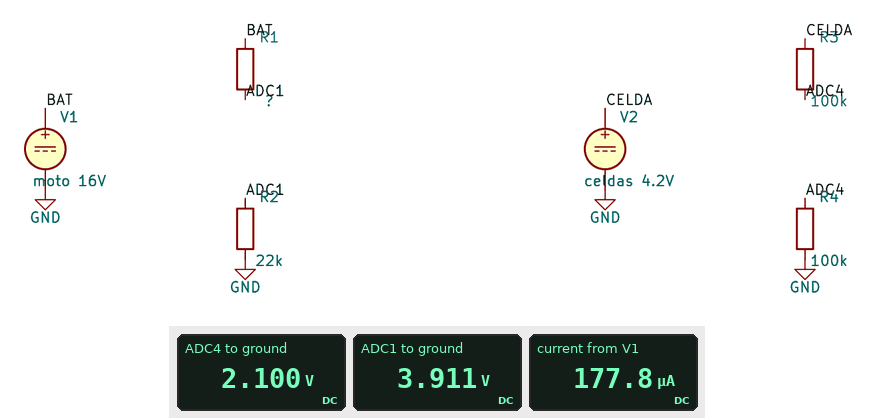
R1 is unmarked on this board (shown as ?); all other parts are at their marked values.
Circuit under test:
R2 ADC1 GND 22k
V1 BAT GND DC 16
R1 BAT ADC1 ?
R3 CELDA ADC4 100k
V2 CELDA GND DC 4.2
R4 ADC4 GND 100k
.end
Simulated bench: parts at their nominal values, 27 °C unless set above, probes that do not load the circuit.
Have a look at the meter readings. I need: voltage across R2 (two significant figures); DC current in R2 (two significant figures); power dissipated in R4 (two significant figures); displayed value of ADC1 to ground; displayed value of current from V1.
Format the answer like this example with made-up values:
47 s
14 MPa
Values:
3.9 V
180 µA
44 µW
3.911 V
177.8 µA
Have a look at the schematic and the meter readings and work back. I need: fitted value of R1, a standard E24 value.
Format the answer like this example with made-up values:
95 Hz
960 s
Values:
68 kΩ
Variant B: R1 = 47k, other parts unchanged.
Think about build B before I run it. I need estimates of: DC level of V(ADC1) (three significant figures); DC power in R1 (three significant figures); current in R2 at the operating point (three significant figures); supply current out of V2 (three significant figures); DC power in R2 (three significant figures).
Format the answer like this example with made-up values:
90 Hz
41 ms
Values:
5.10 V
2.53 mW
232 µA
21.0 µA
1.18 mW
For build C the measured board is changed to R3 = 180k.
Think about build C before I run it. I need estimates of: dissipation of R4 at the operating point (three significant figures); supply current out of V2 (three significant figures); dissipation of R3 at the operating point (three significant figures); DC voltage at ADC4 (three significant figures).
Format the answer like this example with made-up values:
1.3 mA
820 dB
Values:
22.5 µW
15.0 µA
40.5 µW
1.50 V
